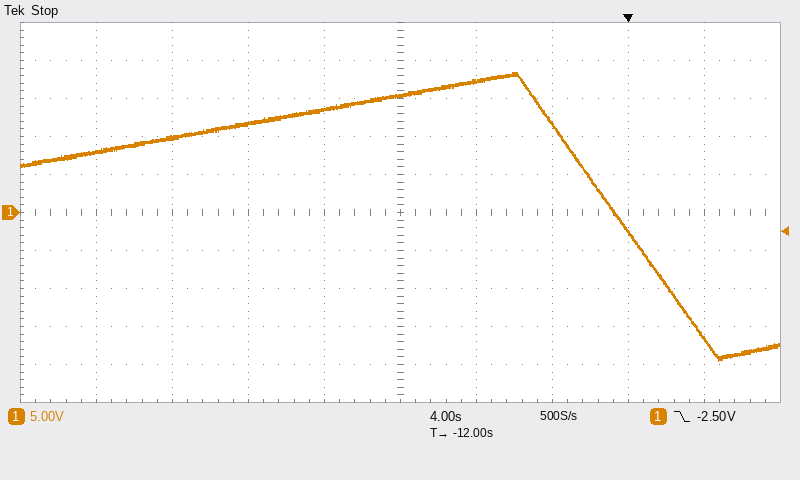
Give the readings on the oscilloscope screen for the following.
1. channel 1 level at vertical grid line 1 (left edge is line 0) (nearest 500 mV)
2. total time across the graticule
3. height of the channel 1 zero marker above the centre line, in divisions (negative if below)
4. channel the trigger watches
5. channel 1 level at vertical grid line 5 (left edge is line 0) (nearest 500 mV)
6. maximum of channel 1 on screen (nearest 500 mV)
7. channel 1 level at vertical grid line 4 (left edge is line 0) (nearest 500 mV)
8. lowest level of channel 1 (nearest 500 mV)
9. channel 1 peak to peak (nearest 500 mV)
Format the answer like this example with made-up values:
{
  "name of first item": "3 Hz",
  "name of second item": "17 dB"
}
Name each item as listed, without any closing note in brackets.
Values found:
{
  "channel 1 level at vertical grid line 1 (left edge is line 0)": "8.0 V",
  "total time across the graticule": "40 s",
  "height of the channel 1 zero marker above the centre line, in divisions": "0.0 div",
  "channel the trigger watches": "channel 1",
  "channel 1 level at vertical grid line 5 (left edge is line 0)": "15.5 V",
  "maximum of channel 1 on screen": "18.5 V",
  "channel 1 level at vertical grid line 4 (left edge is line 0)": "13.5 V",
  "lowest level of channel 1": "-19.5 V",
  "channel 1 peak to peak": "38.0 V"
}
